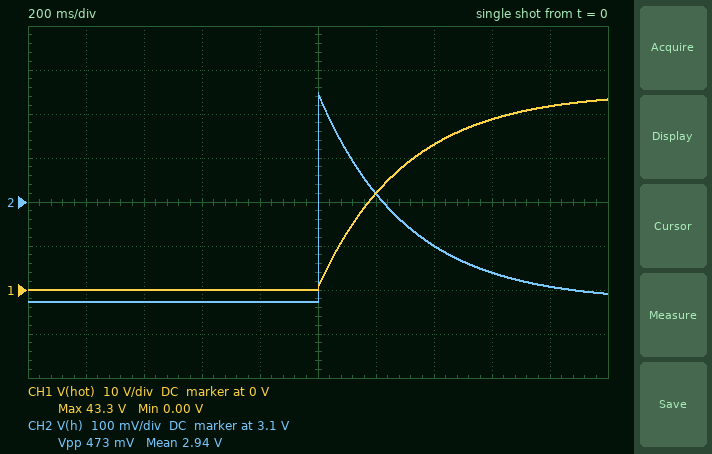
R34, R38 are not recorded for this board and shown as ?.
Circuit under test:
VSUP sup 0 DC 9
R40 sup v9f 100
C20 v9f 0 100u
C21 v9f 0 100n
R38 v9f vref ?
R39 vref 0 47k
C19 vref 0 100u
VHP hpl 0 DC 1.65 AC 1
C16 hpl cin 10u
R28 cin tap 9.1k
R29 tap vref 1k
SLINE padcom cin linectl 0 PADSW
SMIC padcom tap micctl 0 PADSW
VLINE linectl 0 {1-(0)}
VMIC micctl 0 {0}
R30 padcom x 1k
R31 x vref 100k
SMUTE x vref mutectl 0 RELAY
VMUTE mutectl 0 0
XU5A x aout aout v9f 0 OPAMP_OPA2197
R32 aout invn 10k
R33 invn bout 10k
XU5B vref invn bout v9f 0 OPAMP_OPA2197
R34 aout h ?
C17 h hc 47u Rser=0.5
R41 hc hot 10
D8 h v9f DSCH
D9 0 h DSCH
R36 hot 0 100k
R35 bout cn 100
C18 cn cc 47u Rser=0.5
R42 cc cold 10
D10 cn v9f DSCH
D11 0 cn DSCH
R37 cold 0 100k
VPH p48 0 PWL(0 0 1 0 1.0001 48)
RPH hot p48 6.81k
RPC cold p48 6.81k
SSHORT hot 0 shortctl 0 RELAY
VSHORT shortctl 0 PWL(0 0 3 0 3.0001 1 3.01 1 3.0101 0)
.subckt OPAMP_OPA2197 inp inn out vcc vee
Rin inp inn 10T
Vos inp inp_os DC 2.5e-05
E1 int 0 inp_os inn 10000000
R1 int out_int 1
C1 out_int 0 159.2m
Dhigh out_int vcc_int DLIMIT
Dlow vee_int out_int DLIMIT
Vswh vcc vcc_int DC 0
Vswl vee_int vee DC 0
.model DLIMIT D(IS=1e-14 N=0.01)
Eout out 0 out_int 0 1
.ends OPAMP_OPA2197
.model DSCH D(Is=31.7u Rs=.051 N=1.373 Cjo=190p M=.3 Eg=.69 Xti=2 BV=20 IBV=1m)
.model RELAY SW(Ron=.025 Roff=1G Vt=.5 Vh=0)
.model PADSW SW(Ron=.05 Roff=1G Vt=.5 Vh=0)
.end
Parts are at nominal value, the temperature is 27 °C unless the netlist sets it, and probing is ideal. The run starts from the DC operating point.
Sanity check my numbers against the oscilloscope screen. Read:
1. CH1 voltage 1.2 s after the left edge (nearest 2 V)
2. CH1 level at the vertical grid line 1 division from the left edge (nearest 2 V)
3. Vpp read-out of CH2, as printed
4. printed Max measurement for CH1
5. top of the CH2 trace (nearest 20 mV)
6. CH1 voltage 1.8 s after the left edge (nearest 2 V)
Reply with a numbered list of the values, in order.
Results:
1. 22 V
2. 0 V
3. 473 mV
4. 43.3 V
5. 3.34 V
6. 42 V
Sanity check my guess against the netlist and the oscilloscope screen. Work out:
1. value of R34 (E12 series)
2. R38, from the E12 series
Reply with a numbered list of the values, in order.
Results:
1. 68 Ω
2. 100 kΩ
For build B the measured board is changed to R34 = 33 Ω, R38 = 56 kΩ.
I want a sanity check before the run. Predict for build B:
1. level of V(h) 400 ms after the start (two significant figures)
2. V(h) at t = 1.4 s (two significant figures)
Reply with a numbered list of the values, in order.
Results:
1. 4.1 V
2. 4.2 V
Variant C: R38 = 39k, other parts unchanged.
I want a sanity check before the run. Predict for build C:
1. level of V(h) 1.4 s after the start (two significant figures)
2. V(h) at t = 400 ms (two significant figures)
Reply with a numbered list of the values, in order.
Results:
1. 5.0 V
2. 4.9 V
